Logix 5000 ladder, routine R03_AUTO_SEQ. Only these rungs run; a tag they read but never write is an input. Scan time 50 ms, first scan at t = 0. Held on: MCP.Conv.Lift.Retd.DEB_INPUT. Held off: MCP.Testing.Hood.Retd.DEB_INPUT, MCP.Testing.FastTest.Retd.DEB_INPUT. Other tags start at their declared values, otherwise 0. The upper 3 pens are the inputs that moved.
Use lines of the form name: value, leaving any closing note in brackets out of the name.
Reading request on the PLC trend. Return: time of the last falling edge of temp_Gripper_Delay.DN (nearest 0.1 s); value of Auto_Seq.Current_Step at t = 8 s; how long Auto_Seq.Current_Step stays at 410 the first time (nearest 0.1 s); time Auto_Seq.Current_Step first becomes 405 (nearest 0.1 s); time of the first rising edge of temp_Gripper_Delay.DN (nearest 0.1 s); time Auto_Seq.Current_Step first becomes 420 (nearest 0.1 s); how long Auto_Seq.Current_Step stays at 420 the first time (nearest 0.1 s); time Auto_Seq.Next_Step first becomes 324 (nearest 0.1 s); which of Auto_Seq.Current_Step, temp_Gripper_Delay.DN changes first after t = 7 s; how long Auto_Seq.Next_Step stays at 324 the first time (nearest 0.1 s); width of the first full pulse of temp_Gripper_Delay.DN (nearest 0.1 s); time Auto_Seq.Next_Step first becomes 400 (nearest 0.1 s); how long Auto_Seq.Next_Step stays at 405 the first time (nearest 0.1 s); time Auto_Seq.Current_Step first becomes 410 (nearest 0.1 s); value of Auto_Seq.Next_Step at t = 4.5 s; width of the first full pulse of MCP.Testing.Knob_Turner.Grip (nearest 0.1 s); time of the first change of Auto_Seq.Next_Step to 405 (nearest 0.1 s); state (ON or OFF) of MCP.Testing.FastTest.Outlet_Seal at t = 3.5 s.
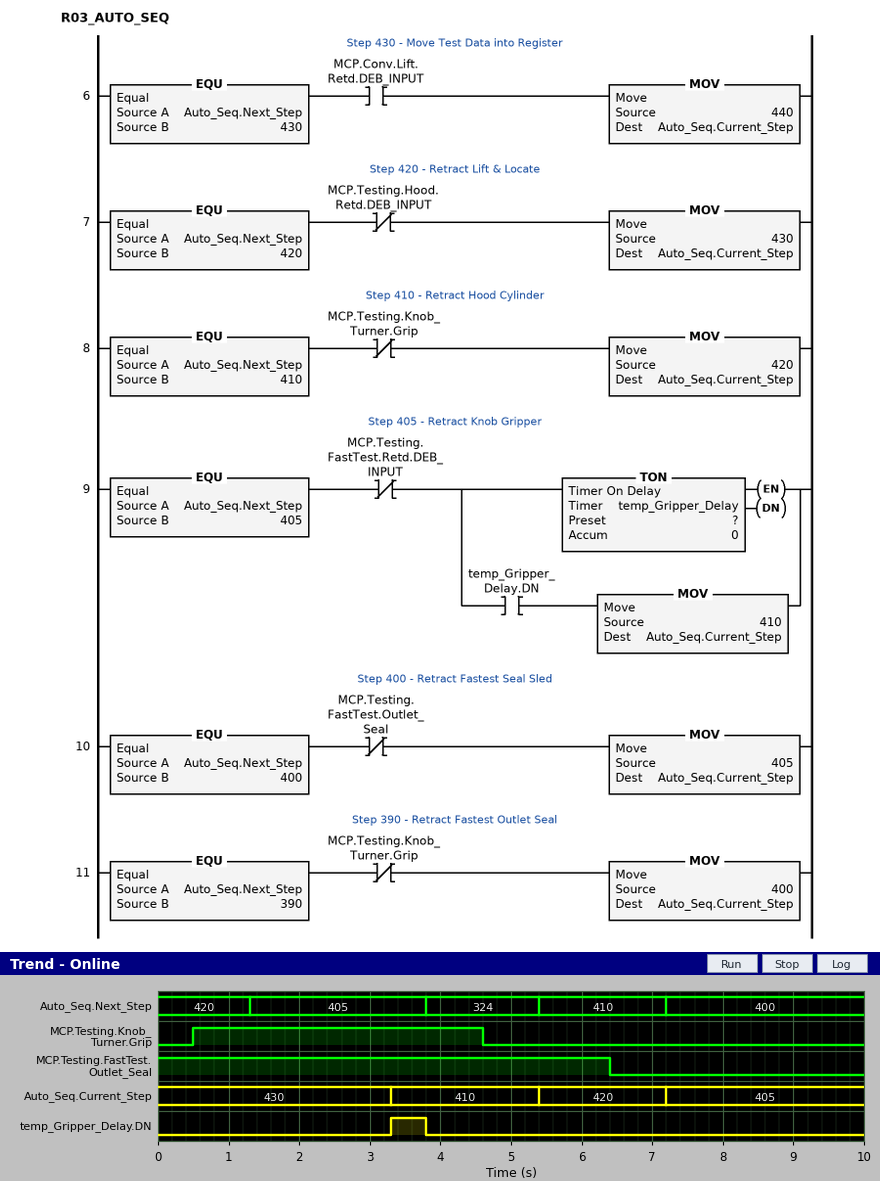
time of the last falling edge of temp_Gripper_Delay.DN: 3.8 s
value of Auto_Seq.Current_Step at t = 8 s: 405
how long Auto_Seq.Current_Step stays at 410 the first time: 2.1 s
time Auto_Seq.Current_Step first becomes 405: 7.2 s
time of the first rising edge of temp_Gripper_Delay.DN: 3.3 s
time Auto_Seq.Current_Step first becomes 420: 5.4 s
how long Auto_Seq.Current_Step stays at 420 the first time: 1.8 s
time Auto_Seq.Next_Step first becomes 324: 3.8 s
which of Auto_Seq.Current_Step, temp_Gripper_Delay.DN changes first after t = 7 s: Auto_Seq.Current_Step
how long Auto_Seq.Next_Step stays at 324 the first time: 1.6 s
width of the first full pulse of temp_Gripper_Delay.DN: 0.5 s
time Auto_Seq.Next_Step first becomes 400: 7.2 s
how long Auto_Seq.Next_Step stays at 405 the first time: 2.5 s
time Auto_Seq.Current_Step first becomes 410: 3.3 s
value of Auto_Seq.Next_Step at t = 4.5 s: 324
width of the first full pulse of MCP.Testing.Knob_Turner.Grip: 4.1 s
time of the first change of Auto_Seq.Next_Step to 405: 1.3 s
state (ON or OFF) of MCP.Testing.FastTest.Outlet_Seal at t = 3.5 s: ON
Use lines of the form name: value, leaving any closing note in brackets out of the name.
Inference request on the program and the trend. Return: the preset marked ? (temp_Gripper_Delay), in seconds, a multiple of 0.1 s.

the preset marked ? (temp_Gripper_Delay), in seconds, a multiple of 0.1 s: 2.0 s
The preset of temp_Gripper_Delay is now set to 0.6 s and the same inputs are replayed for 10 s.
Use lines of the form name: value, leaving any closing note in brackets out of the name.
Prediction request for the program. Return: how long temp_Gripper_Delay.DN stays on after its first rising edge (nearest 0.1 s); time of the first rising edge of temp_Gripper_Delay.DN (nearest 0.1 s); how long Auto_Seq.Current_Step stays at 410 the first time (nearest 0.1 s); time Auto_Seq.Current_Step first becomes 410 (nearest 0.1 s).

how long temp_Gripper_Delay.DN stays on after its first rising edge: 1.9 s
time of the first rising edge of temp_Gripper_Delay.DN: 1.9 s
how long Auto_Seq.Current_Step stays at 410 the first time: 3.5 s
time Auto_Seq.Current_Step first becomes 410: 1.9 s
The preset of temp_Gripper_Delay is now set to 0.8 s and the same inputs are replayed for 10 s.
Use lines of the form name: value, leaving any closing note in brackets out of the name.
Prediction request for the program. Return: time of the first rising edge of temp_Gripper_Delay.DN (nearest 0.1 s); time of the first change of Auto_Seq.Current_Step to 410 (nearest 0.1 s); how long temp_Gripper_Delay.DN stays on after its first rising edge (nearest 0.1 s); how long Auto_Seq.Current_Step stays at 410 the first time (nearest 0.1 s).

time of the first rising edge of temp_Gripper_Delay.DN: 2.1 s
time of the first change of Auto_Seq.Current_Step to 410: 2.1 s
how long temp_Gripper_Delay.DN stays on after its first rising edge: 1.7 s
how long Auto_Seq.Current_Step stays at 410 the first time: 3.3 s
